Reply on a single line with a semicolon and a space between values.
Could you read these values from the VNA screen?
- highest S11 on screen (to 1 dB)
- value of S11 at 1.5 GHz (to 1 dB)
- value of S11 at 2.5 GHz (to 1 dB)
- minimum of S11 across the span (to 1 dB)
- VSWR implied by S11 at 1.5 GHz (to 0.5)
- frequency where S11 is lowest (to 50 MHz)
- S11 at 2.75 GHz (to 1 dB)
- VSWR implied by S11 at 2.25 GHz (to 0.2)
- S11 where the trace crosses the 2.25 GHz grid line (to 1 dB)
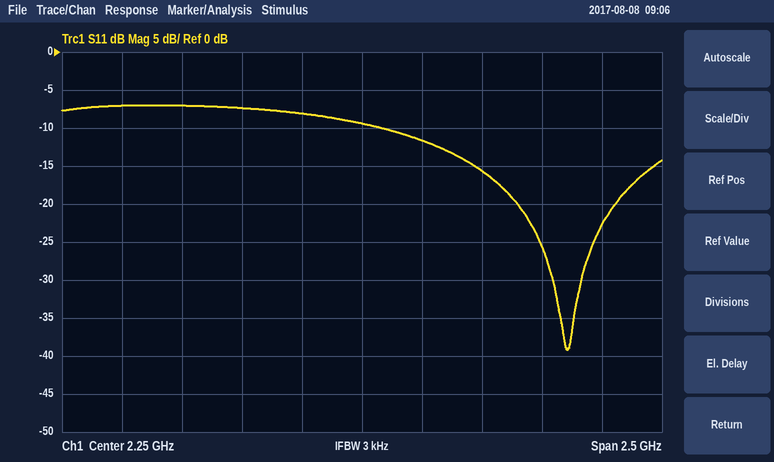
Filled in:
-7 dB; -7 dB; -12 dB; -39 dB; 2.5; 3.10 GHz; -16 dB; 2.0; -9 dB
